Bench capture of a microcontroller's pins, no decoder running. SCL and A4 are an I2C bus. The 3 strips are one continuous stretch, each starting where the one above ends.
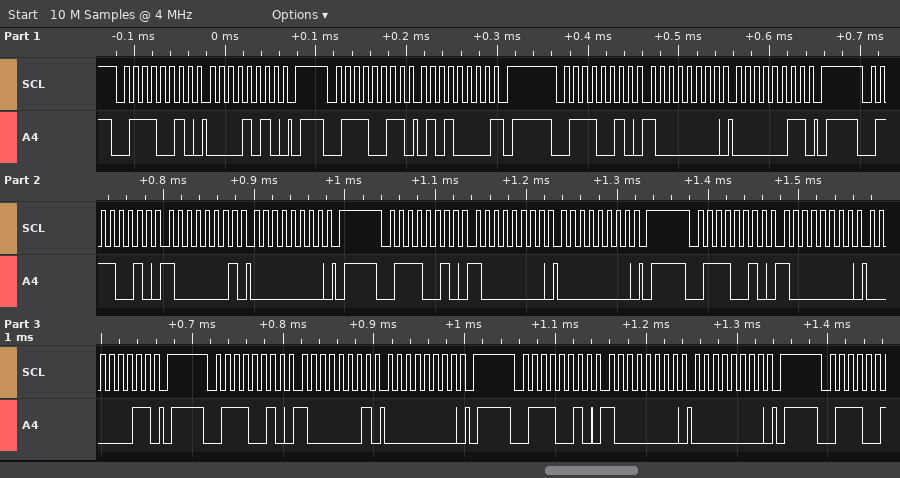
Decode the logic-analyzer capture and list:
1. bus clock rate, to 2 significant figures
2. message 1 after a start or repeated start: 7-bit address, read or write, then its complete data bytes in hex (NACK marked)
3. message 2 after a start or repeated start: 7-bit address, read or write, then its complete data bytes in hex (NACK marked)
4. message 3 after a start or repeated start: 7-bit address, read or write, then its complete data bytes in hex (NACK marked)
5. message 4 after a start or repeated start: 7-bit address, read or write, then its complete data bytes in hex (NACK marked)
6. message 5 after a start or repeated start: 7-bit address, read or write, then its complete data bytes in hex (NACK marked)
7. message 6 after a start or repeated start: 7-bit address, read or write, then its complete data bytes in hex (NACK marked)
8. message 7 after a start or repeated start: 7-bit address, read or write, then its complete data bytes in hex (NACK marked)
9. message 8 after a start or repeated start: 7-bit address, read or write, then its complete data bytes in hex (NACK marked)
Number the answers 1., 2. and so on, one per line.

1. 100 kHz
2. 0x39 write: 0A
3. 0x39 read: 50 NACK
4. 0x39 write: 80 03
5. 0x39 write: 81 00
6. 0x39 write: 80 00
7. 0x39 write: 80 03
8. 0x39 write: 81 00
9. 0x39 write: 80 00
